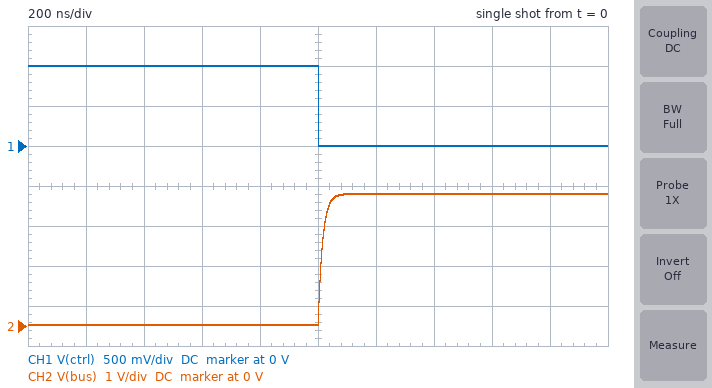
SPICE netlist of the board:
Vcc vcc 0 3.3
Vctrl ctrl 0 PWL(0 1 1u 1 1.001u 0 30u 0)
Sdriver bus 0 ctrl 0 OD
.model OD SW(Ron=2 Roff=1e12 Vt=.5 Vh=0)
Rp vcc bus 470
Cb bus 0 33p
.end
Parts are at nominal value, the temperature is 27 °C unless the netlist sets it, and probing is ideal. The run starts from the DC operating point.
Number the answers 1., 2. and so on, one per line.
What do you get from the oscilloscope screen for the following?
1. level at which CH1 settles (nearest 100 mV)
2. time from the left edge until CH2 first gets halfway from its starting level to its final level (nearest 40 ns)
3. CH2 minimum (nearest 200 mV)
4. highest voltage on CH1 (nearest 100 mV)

1. 0 V
2. 1.00 µs
3. 0 V
4. 1.0 V
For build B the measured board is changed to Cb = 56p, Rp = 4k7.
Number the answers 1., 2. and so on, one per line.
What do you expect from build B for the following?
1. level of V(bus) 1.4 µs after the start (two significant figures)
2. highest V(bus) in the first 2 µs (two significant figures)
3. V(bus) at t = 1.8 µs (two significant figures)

1. 2.6 V
2. 3.2 V
3. 3.1 V
